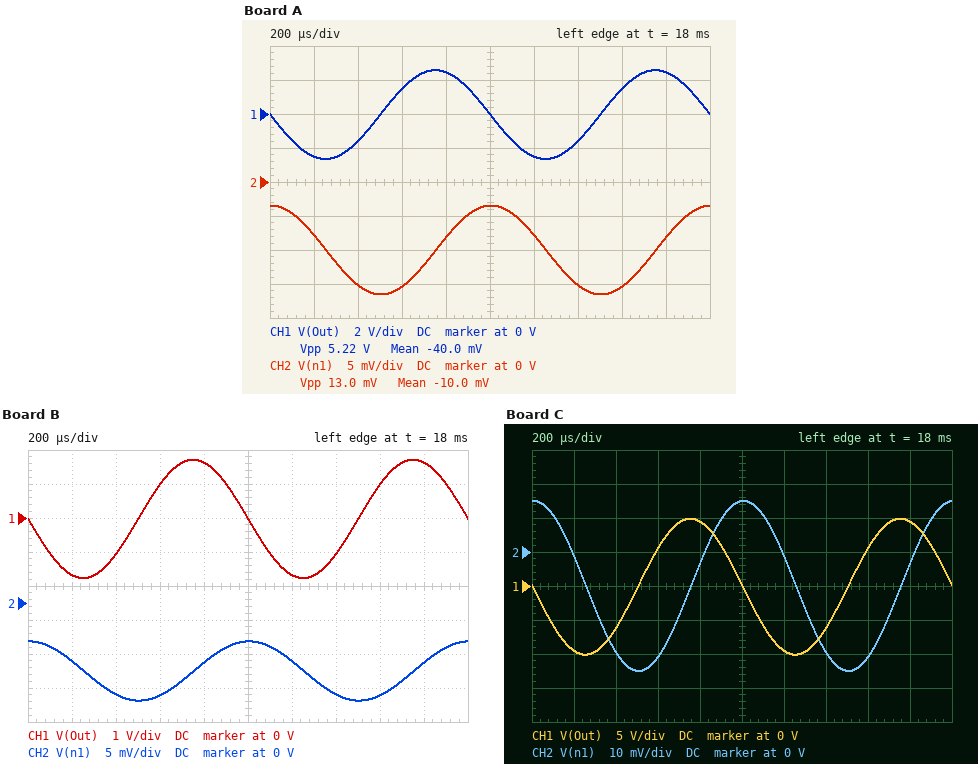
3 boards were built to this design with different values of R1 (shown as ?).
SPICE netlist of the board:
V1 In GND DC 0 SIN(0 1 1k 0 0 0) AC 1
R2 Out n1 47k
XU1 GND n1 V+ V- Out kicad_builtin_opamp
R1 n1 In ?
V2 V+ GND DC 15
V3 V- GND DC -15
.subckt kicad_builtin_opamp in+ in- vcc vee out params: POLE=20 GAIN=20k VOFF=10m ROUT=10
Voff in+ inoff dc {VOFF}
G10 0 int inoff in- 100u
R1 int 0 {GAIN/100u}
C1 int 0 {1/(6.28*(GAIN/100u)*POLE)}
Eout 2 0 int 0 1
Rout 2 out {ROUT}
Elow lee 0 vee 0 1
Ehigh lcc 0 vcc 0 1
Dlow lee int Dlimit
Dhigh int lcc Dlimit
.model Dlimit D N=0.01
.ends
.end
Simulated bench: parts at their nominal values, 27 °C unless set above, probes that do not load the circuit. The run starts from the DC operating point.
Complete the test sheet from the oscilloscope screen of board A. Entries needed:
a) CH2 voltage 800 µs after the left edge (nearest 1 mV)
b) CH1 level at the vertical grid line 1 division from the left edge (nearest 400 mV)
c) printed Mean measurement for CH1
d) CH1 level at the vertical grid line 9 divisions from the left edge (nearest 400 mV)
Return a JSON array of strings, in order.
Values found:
["-8 mV", "-2.4 V", "-40.0 mV", "2.4 V"]
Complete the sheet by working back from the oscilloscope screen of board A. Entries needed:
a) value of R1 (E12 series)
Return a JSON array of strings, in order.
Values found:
["18 kΩ"]
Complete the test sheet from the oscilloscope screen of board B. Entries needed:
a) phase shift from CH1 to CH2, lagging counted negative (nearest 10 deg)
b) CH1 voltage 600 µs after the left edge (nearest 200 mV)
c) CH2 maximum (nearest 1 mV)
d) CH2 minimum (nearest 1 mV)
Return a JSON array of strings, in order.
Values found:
["-90 deg", "1.0 V", "-6 mV", "-14 mV"]
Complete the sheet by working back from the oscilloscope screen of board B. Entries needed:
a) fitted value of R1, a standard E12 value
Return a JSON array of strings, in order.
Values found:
["27 kΩ"]
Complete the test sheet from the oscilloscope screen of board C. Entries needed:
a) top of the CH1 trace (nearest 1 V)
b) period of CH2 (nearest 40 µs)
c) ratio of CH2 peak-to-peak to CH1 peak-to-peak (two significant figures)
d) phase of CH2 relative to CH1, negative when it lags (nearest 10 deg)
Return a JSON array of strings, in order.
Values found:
["10 V", "1.00 ms", "0.0025", "-90 deg"]
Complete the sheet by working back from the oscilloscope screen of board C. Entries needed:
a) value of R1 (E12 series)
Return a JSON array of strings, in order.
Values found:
["4.7 kΩ"]
